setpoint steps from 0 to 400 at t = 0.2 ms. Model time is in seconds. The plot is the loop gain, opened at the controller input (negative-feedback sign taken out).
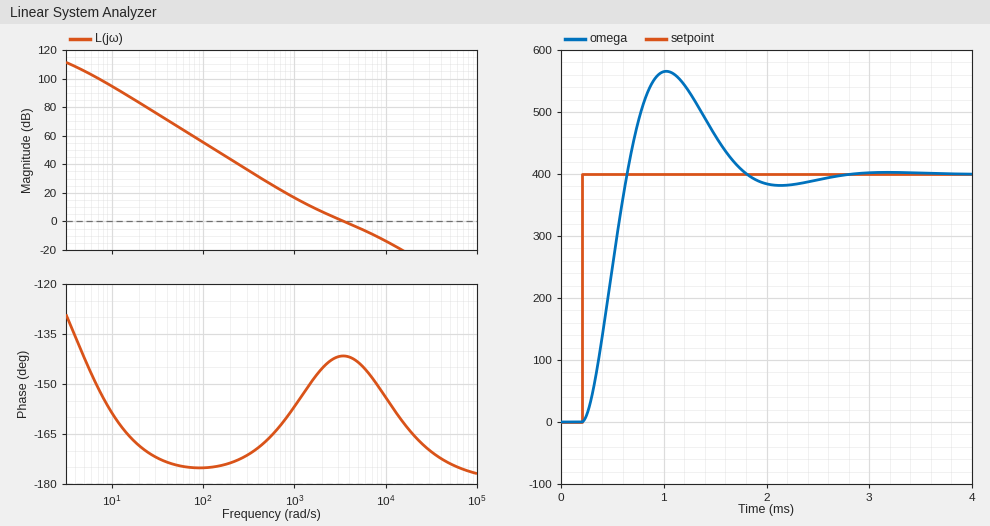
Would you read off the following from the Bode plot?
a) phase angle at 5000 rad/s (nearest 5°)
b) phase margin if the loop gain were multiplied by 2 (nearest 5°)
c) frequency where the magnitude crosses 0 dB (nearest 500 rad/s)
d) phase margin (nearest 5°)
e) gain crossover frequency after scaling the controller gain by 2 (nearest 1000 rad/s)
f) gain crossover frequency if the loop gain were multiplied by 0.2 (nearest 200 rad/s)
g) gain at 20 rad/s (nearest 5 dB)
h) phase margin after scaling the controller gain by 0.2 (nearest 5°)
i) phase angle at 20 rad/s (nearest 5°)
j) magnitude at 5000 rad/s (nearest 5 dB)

-145°
35°
3500 rad/s
40°
6000 rad/s
1200 rad/s
85 dB
25°
-170°
-5 dB
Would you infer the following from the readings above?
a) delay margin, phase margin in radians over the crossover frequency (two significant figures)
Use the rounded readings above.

0.00020 s
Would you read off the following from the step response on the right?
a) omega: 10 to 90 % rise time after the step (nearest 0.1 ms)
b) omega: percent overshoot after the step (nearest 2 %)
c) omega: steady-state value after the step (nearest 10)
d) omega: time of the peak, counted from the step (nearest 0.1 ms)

0.3 ms
42 %
400
0.8 ms
